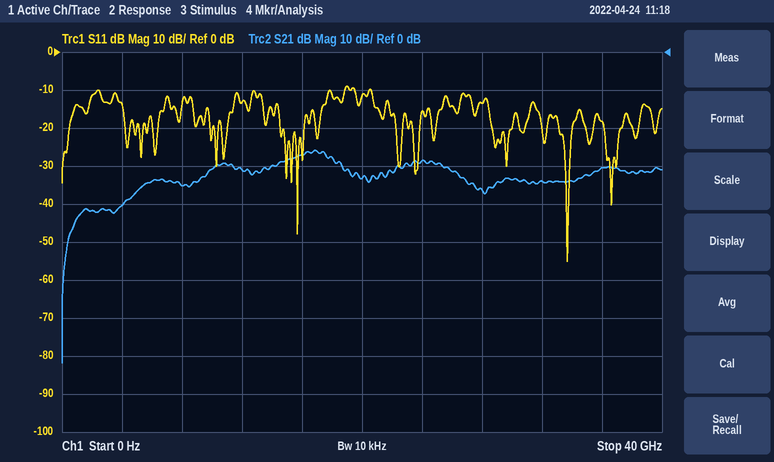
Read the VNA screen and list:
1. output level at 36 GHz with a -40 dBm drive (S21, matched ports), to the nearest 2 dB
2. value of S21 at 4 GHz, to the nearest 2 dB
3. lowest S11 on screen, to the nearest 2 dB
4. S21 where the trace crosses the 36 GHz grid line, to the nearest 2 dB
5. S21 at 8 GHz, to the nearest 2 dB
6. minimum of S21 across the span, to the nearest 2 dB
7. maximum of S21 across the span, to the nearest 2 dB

-70 dBm
-40 dB
-56 dB
-30 dB
-36 dB
-82 dB
-26 dB
